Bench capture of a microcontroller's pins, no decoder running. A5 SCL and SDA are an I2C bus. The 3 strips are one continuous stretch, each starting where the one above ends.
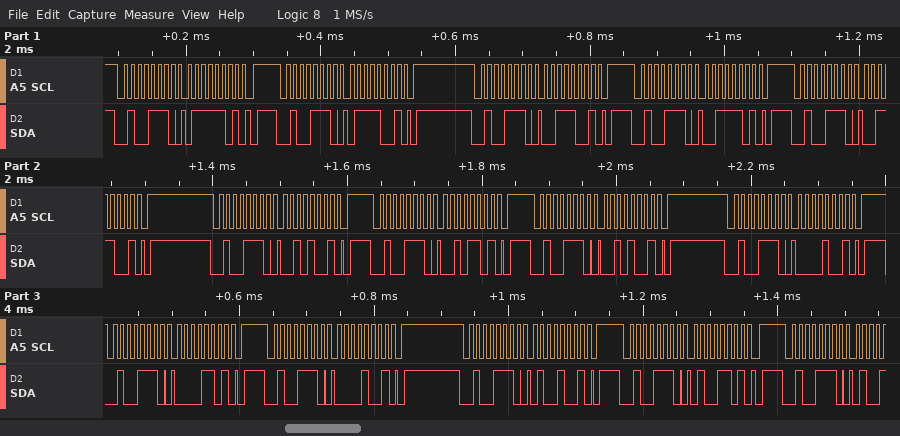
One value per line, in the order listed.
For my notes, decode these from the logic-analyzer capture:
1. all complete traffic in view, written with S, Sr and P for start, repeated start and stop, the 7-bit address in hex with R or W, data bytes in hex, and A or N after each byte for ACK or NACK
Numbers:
S 27W A 7D A P S 27W A 79 A P S 27W A 39 A P S 27W A 3D A P S 27W A 39 A P S 27W A 29 A P S 27W A 2D A P S 27W A 29 A P S 27W A 09 A P S 27W A 0D A P S 27W A 09 A P S 27W A 49 A P S 27W A 4D A P S 27W A
